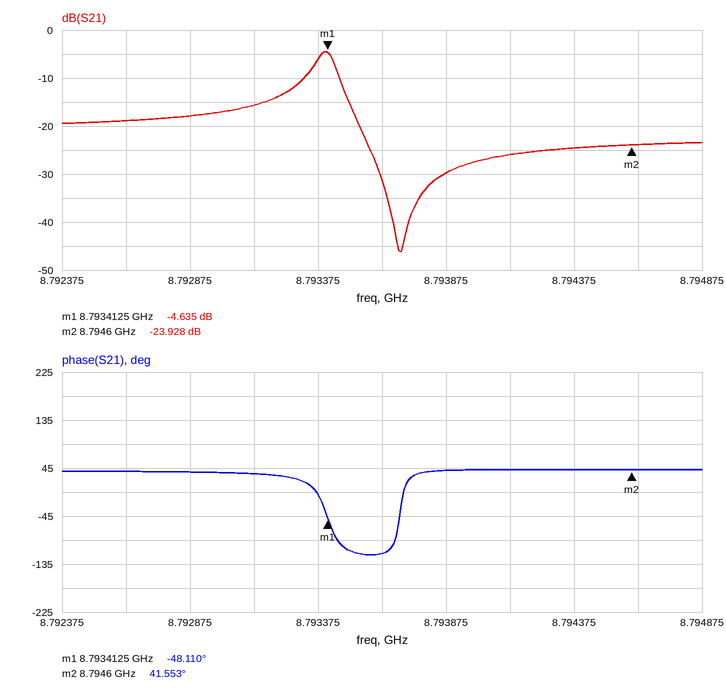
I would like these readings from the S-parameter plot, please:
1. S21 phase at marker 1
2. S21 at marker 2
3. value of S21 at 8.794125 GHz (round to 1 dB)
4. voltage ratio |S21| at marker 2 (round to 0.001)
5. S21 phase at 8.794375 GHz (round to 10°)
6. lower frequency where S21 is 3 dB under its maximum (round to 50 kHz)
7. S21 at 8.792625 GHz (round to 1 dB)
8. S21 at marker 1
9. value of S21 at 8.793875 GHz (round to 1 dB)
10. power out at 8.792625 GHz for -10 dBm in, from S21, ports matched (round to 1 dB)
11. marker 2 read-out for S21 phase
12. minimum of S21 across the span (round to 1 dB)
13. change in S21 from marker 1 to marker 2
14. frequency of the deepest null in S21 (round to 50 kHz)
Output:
-48.110°
-23.928 dB
-26 dB
0.064
40°
8.79335 GHz
-19 dB
-4.635 dB
-30 dB
-29 dBm
41.553°
-46 dB
-19.293 dB
8.79370 GHz
